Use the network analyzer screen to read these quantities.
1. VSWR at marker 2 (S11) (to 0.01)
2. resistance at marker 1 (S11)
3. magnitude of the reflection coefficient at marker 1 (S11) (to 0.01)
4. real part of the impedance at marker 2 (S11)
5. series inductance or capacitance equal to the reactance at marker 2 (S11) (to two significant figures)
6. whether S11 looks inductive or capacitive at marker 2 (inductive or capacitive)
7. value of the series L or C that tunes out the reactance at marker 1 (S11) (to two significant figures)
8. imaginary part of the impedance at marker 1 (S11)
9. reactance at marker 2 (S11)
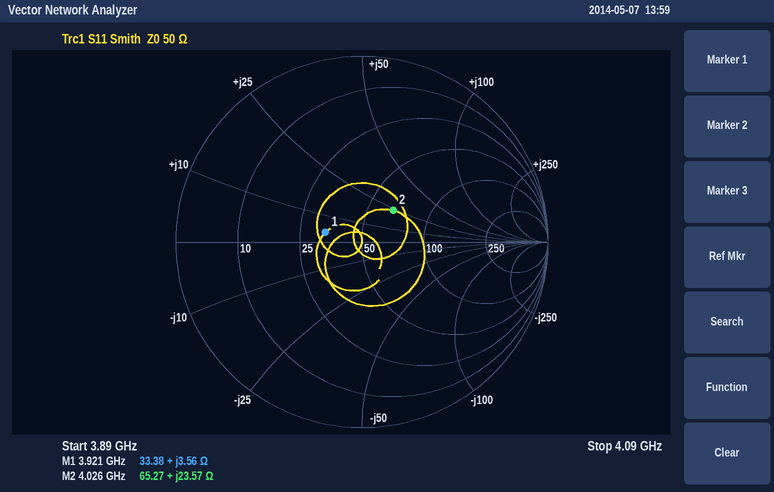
1.63
33.38 Ω
0.20
65.27 Ω
930 pH
inductive
11 pF
+3.56 Ω
+23.57 Ω
